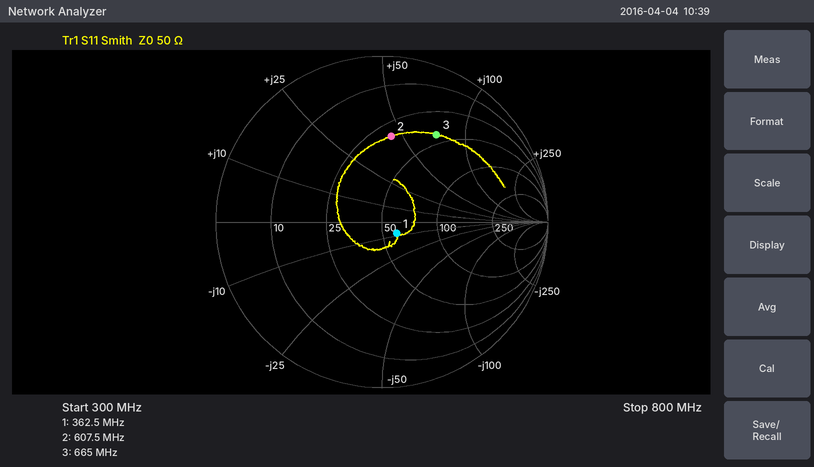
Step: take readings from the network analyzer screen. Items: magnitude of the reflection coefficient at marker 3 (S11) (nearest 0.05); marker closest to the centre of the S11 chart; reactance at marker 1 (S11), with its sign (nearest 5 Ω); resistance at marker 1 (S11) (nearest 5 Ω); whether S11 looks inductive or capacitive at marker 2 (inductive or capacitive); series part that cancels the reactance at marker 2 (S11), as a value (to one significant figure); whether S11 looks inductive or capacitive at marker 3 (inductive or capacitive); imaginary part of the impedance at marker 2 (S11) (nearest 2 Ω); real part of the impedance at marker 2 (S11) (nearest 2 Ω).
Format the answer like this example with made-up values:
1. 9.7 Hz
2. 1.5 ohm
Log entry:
1. 0.60
2. marker 1
3. -10 Ω
4. 60 Ω
5. inductive
6. 6 pF
7. inductive
8. +44 Ω
9. 32 Ω
